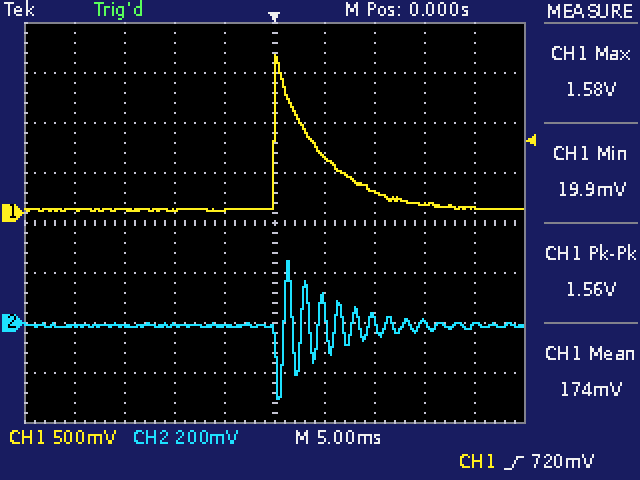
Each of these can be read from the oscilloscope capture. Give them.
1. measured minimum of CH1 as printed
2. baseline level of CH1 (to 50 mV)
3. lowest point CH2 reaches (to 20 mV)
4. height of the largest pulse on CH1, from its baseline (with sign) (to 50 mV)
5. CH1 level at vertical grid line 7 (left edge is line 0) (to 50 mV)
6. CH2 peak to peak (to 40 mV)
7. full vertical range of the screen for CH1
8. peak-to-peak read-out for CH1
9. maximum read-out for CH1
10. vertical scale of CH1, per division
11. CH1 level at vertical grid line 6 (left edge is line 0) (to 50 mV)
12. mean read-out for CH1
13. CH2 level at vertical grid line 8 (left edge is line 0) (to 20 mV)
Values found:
19.9 mV
50 mV
-300 mV
+1.55 V
200 mV
560 mV
4 V
1.56 V
1.58 V
500 mV
550 mV
174 mV
0 mV
